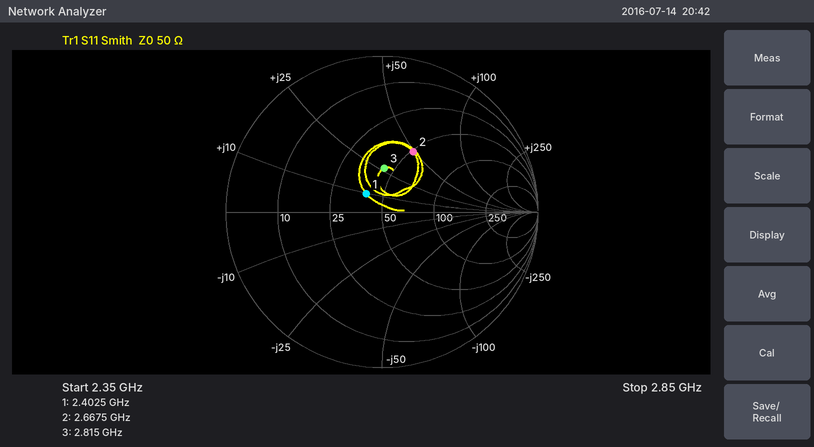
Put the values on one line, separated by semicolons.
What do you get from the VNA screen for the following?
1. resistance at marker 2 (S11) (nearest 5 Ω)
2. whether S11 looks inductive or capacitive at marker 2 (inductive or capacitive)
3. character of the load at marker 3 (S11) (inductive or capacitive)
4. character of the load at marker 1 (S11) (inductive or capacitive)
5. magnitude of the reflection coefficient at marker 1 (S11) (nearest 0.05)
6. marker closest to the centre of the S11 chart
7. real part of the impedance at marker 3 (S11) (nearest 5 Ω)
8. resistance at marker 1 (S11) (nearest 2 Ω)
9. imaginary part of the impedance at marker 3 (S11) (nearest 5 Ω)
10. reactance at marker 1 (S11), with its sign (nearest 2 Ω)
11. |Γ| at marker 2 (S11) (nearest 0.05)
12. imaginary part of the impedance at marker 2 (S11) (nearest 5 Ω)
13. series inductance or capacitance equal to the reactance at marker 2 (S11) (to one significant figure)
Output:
50 Ω; inductive; inductive; inductive; 0.15; marker 1; 45 Ω; 40 Ω; +25 Ω; +10 Ω; 0.45; +50 Ω; 3 nH
